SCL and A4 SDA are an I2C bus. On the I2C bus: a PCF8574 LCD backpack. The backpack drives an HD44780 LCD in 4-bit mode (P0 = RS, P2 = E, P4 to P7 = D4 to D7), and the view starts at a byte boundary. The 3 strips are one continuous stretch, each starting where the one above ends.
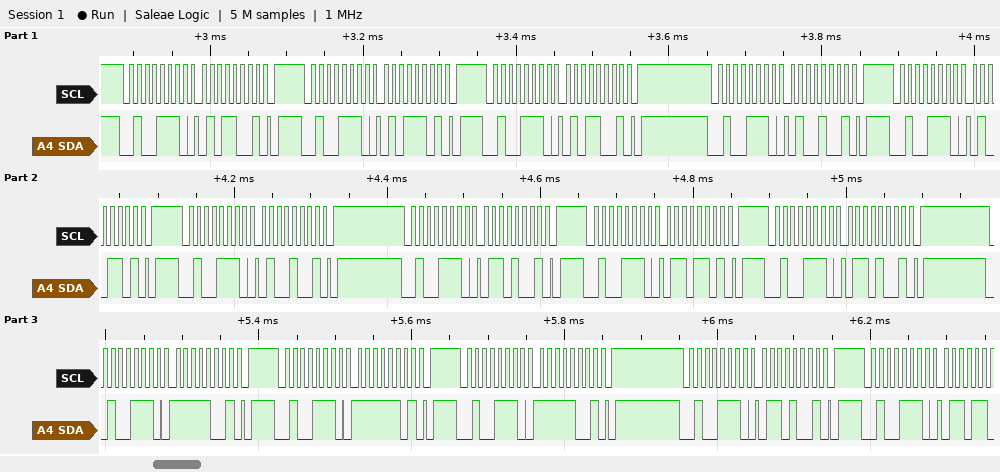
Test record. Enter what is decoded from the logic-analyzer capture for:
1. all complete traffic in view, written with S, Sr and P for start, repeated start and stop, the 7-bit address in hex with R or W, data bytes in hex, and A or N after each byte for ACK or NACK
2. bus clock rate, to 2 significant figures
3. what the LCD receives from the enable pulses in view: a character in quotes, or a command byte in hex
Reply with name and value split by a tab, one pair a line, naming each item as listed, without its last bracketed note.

all complete traffic in view, written with S, Sr and P for start, repeated start and stop, the 7-bit address in hex with R or W, data bytes in hex, and A or N after each byte for ACK or NACK	S 27W A 59 A P S 27W A 5D A P S 27W A 59 A P S 27W A 49 A P S 27W A 4D A P S 27W A 49 A P S 27W A 69 A P S 27W A 6D A P S 27W A 69 A P S 27W A F9 A P S 27W A FD A P S 27W A F9 A P S 27W A 69 A P S 27W A
bus clock rate, to 2 significant figures	100 kHz
what the LCD receives from the enable pulses in view: a character in quotes, or a command byte in hex	'T' 'o'
